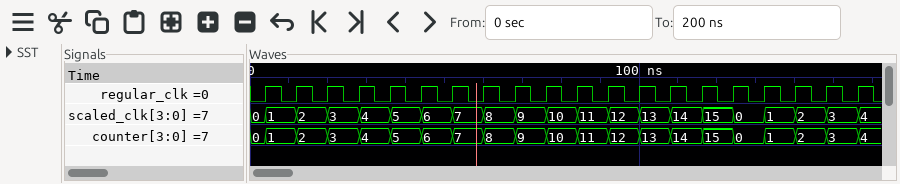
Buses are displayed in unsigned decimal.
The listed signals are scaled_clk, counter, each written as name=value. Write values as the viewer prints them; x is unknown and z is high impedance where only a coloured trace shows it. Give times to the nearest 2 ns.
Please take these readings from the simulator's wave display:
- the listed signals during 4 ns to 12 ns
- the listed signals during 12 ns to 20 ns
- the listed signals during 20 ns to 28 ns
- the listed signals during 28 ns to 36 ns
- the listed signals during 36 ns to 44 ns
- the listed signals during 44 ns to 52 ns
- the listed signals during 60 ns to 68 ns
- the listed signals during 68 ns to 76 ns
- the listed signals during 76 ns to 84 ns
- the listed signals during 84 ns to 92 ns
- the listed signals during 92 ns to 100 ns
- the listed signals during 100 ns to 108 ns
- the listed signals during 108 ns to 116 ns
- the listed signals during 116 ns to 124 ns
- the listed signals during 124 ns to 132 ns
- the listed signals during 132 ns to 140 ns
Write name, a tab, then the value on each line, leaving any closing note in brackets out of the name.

the listed signals during 4 ns to 12 ns	scaled_clk=1, counter=1
the listed signals during 12 ns to 20 ns	scaled_clk=2, counter=2
the listed signals during 20 ns to 28 ns	scaled_clk=3, counter=3
the listed signals during 28 ns to 36 ns	scaled_clk=4, counter=4
the listed signals during 36 ns to 44 ns	scaled_clk=5, counter=5
the listed signals during 44 ns to 52 ns	scaled_clk=6, counter=6
the listed signals during 60 ns to 68 ns	scaled_clk=8, counter=8
the listed signals during 68 ns to 76 ns	scaled_clk=9, counter=9
the listed signals during 76 ns to 84 ns	scaled_clk=10, counter=10
the listed signals during 84 ns to 92 ns	scaled_clk=11, counter=11
the listed signals during 92 ns to 100 ns	scaled_clk=12, counter=12
the listed signals during 100 ns to 108 ns	scaled_clk=13, counter=13
the listed signals during 108 ns to 116 ns	scaled_clk=14, counter=14
the listed signals during 116 ns to 124 ns	scaled_clk=15, counter=15
the listed signals during 124 ns to 132 ns	scaled_clk=0, counter=0
the listed signals during 132 ns to 140 ns	scaled_clk=1, counter=1
